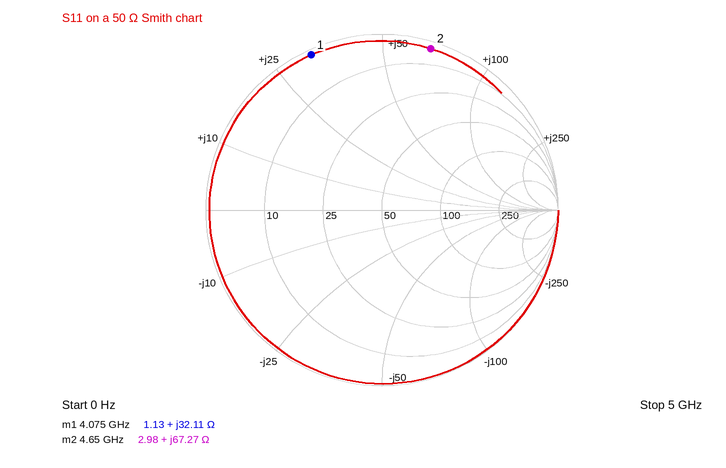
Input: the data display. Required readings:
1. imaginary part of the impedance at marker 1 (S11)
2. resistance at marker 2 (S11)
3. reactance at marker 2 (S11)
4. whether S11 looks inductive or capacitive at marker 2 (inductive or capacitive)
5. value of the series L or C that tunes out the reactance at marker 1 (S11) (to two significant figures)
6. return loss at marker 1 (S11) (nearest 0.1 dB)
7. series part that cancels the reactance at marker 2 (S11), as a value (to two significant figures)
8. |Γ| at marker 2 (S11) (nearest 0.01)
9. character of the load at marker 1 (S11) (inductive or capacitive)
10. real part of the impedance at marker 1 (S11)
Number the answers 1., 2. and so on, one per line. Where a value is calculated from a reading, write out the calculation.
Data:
1. +32.11 Ω
2. 2.98 Ω
3. +67.27 Ω
4. inductive
5. C = 1/(2π × 4.075 GHz × 32.11 Ω) ≈ 1.2 pF
6. 0.3 dB
7. C = 1/(2π × 4.65 GHz × 67.27 Ω) ≈ 509 fF, so 510 fF to two significant figures
8. 0.96
9. inductive
10. 1.13 Ω
